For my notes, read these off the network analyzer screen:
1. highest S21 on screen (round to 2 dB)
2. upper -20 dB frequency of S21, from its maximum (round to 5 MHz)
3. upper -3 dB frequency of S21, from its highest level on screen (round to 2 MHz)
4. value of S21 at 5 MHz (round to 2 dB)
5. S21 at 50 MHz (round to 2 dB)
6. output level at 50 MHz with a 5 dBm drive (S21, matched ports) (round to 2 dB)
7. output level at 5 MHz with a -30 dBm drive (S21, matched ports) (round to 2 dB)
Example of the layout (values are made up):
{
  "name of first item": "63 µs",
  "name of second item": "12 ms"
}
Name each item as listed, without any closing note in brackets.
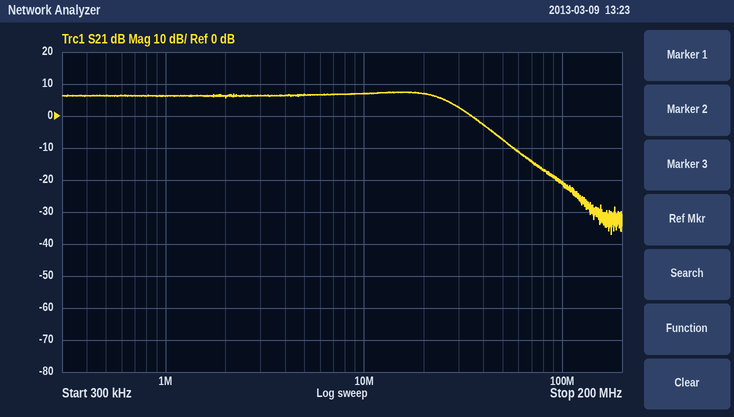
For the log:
{
  "highest S21 on screen": "8 dB",
  "upper -20 dB frequency of S21, from its maximum": "65 MHz",
  "upper -3 dB frequency of S21, from its highest level on screen": "26 MHz",
  "value of S21 at 5 MHz": "6 dB",
  "S21 at 50 MHz": "-8 dB",
  "output level at 50 MHz with a 5 dBm drive (S21, matched ports)": "-2 dBm",
  "output level at 5 MHz with a -30 dBm drive (S21, matched ports)": "-24 dBm"
}
